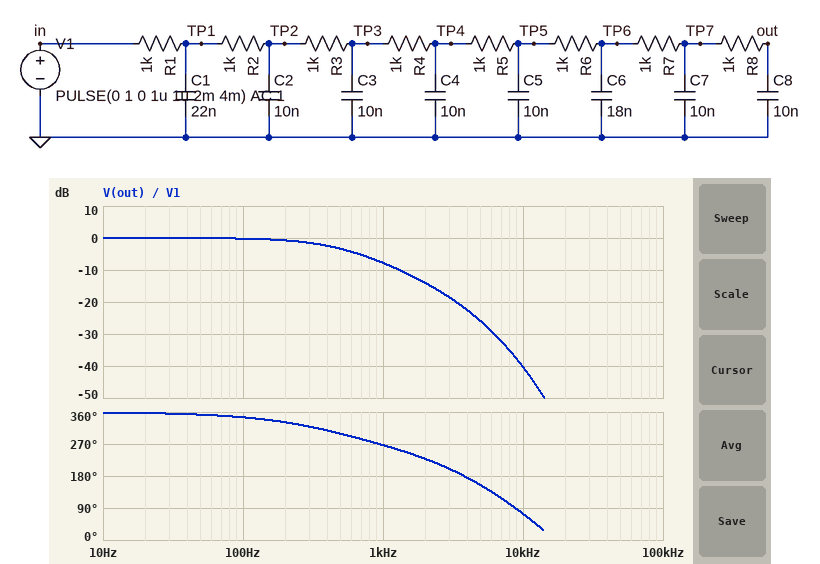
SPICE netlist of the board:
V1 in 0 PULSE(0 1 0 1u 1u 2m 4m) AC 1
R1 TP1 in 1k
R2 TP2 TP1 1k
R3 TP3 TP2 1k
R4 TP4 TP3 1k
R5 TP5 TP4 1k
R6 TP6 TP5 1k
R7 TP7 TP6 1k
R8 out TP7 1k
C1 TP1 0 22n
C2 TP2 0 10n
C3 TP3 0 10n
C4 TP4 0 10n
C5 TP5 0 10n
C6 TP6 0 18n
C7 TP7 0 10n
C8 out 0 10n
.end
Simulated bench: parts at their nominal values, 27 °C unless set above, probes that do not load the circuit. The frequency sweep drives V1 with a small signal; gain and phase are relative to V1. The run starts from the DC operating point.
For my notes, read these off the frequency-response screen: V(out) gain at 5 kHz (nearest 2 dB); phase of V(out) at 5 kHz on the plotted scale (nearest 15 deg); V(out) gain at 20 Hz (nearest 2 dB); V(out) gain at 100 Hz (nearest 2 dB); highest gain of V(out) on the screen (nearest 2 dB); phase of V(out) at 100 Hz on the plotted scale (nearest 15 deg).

-26 dB
150 deg
0 dB
0 dB
0 dB
345 deg
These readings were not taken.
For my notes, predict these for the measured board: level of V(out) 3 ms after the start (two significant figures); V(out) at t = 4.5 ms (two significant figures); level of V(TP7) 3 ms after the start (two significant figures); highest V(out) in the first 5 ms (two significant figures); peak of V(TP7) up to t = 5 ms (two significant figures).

68 mV
710 mV
66 mV
1.0 V
1.0 V
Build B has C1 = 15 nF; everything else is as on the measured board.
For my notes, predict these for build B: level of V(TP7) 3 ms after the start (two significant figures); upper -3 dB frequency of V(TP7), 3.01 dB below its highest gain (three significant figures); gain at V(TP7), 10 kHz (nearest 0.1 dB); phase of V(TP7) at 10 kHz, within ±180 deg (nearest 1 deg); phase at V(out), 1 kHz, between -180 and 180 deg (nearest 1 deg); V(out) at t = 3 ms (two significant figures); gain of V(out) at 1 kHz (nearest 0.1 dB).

64 mV
463 Hz
-37.6 dB
115 deg
-91 deg
66 mV
-7.7 dB
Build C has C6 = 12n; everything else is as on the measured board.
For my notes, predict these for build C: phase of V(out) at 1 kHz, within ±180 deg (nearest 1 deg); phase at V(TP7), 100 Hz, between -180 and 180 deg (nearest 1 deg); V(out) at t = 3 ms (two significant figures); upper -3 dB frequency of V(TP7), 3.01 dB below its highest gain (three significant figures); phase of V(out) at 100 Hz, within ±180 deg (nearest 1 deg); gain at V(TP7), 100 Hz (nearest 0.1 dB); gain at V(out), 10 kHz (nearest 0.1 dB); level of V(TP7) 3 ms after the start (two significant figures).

-90 deg
-13 deg
50 mV
509 Hz
-14 deg
-0.2 dB
-38.9 dB
49 mV
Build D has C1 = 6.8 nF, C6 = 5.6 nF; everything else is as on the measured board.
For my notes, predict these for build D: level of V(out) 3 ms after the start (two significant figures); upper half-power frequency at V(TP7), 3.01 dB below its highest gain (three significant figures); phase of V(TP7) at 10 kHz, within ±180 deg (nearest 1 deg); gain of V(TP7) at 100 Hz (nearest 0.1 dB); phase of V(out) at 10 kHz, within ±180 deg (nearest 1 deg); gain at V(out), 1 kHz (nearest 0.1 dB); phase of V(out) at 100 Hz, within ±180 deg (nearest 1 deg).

31 mV
583 Hz
144 deg
-0.1 dB
112 deg
-6.1 dB
-12 deg
